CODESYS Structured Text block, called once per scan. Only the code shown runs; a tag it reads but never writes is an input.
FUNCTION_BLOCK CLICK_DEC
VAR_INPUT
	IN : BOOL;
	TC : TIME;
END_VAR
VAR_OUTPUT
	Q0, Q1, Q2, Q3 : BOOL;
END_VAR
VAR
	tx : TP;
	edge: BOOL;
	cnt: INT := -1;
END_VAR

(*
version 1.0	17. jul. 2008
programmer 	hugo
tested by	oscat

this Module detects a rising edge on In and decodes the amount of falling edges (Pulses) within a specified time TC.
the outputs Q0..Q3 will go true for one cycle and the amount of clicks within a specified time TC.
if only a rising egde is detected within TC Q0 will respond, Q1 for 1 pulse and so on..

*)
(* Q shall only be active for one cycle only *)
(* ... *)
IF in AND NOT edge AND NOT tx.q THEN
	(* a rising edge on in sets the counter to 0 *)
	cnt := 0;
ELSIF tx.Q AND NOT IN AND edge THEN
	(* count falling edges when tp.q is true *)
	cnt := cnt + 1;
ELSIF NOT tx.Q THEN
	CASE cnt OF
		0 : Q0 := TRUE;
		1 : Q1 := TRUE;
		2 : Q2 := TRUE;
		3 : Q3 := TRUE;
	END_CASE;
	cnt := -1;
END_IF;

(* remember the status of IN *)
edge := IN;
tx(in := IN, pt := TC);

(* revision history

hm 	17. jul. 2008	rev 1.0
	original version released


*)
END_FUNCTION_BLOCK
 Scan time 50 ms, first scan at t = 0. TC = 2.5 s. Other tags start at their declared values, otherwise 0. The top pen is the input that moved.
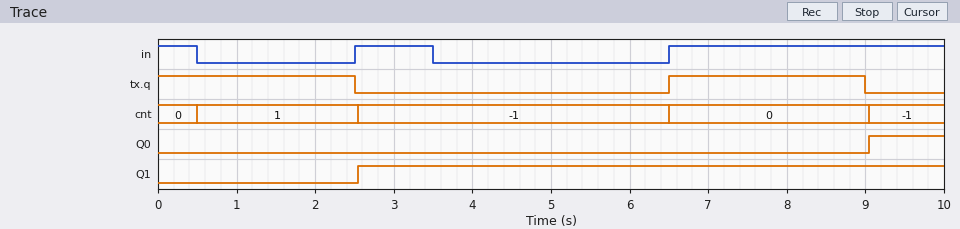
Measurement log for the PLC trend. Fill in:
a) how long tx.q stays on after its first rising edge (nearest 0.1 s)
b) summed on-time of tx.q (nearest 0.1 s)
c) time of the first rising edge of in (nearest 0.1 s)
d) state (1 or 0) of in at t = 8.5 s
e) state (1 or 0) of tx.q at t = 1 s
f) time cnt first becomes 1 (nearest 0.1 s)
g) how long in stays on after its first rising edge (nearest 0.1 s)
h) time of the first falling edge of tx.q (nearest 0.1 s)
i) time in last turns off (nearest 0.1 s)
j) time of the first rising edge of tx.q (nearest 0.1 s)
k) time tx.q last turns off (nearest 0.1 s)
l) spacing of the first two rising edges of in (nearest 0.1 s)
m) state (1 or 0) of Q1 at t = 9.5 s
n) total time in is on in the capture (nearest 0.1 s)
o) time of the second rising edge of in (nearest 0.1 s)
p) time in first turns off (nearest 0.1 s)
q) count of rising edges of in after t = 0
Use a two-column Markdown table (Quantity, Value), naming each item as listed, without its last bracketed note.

| Quantity | Value |
|---|---|
| how long tx.q stays on after its first rising edge | 2.5 s |
| summed on-time of tx.q | 5.0 s |
| time of the first rising edge of in | 2.5 s |
| state (1 or 0) of in at t = 8.5 s | 1 |
| state (1 or 0) of tx.q at t = 1 s | 1 |
| time cnt first becomes 1 | 0.5 s |
| how long in stays on after its first rising edge | 1.0 s |
| time of the first falling edge of tx.q | 2.5 s |
| time in last turns off | 3.5 s |
| time of the first rising edge of tx.q | 6.5 s |
| time tx.q last turns off | 9.0 s |
| spacing of the first two rising edges of in | 4.0 s |
| state (1 or 0) of Q1 at t = 9.5 s | 1 |
| total time in is on in the capture | 5.0 s |
| time of the second rising edge of in | 6.5 s |
| time in first turns off | 0.5 s |
| count of rising edges of in after t = 0 | 2 |
